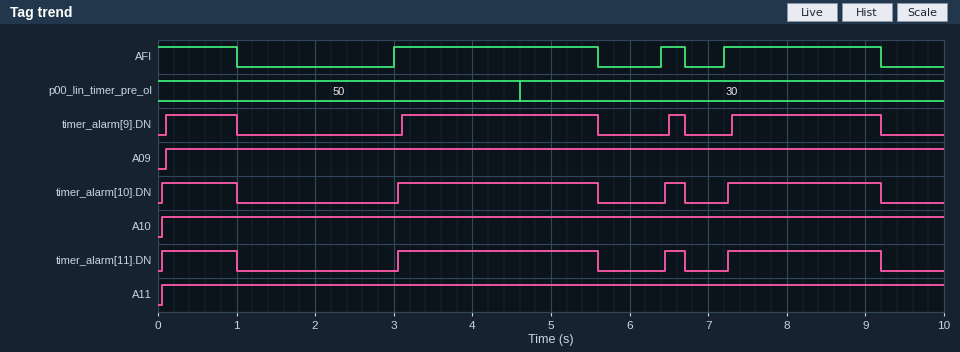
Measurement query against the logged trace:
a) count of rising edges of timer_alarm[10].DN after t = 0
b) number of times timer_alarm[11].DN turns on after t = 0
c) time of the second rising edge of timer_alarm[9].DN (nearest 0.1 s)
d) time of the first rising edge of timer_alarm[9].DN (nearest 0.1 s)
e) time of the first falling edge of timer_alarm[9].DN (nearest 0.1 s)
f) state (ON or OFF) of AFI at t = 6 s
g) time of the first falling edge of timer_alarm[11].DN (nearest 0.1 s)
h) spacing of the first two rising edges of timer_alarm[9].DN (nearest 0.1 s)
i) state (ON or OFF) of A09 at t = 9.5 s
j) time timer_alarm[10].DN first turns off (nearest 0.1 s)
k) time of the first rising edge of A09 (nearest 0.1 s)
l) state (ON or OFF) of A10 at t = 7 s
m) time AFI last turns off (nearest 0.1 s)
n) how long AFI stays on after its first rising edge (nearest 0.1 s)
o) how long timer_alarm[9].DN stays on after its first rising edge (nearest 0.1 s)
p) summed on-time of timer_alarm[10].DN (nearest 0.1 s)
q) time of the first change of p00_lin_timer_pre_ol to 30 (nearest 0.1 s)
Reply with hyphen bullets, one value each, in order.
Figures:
- 4
- 4
- 3.1 s
- 0.1 s
- 1.0 s
- OFF
- 1.0 s
- 3.0 s
- ON
- 1.0 s
- 0.1 s
- ON
- 9.2 s
- 2.6 s
- 0.9 s
- 5.7 s
- 4.6 s
